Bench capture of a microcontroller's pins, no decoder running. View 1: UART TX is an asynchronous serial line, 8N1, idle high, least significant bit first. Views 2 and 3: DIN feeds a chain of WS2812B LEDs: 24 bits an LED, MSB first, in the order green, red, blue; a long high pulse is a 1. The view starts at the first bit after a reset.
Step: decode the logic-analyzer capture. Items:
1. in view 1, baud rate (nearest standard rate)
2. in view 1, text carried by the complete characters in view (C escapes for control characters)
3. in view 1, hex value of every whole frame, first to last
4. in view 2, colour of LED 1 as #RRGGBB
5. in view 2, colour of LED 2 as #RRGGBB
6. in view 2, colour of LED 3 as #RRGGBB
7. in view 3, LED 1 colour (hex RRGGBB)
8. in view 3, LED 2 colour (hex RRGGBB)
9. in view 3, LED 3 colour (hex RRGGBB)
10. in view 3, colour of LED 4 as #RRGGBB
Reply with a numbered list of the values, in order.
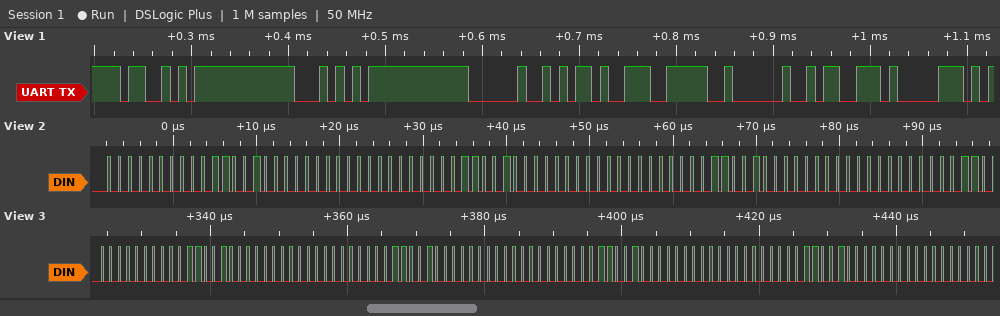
1. 115200 baud
2. "ST -> sp"
3. 53 54 20 2D 3E 20 73 70
4. #320000
5. #320000
6. #320000
7. #320000
8. #320000
9. #320000
10. #320000
